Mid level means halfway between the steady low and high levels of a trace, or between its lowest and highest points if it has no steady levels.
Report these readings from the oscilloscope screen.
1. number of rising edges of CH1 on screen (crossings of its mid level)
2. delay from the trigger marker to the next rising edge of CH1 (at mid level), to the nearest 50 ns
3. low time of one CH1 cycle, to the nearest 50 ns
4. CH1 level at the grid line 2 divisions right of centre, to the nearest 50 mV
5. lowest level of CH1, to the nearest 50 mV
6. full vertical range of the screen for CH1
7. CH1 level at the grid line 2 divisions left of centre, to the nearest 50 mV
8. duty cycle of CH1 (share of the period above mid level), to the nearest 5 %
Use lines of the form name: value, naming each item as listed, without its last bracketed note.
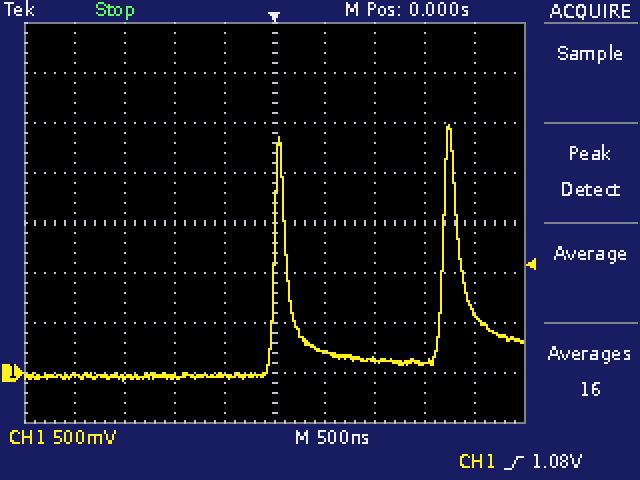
number of rising edges of CH1 on screen: 2
delay from the trigger marker to the next rising edge of CH1 (at mid level), to the nearest 50 ns: 1.70 µs
low time of one CH1 cycle, to the nearest 50 ns: 1.55 µs
CH1 level at the grid line 2 divisions right of centre, to the nearest 50 mV: 150 mV
lowest level of CH1, to the nearest 50 mV: -100 mV
full vertical range of the screen for CH1: 4 V
CH1 level at the grid line 2 divisions left of centre, to the nearest 50 mV: -50 mV
duty cycle of CH1 (share of the period above mid level), to the nearest 5 %: 10 %
